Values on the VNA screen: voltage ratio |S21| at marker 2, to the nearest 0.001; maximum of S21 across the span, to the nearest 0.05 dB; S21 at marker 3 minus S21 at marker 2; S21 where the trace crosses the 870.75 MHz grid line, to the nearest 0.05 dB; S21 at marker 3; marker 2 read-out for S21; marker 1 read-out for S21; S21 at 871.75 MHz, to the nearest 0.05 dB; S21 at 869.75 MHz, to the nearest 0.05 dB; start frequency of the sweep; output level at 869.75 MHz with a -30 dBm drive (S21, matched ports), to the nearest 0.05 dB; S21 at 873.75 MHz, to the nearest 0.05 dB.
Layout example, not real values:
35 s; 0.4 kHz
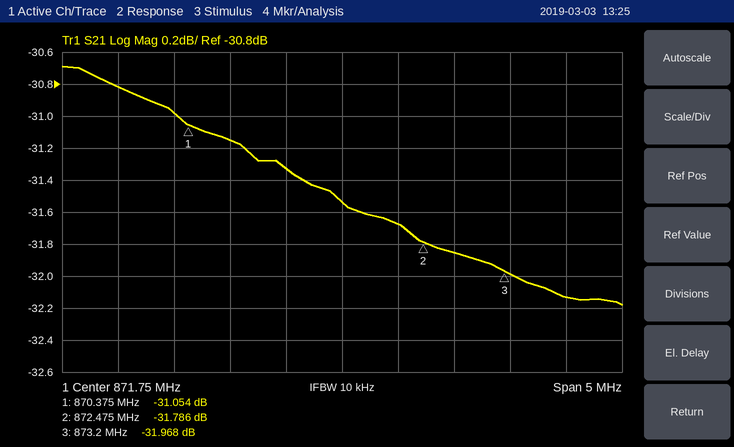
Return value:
0.026; -30.70 dB; -0.182 dB; -31.15 dB; -31.968 dB; -31.786 dB; -31.054 dB; -31.55 dB; -30.80 dB; 869.25 MHz; -60.80 dBm; -32.15 dB
